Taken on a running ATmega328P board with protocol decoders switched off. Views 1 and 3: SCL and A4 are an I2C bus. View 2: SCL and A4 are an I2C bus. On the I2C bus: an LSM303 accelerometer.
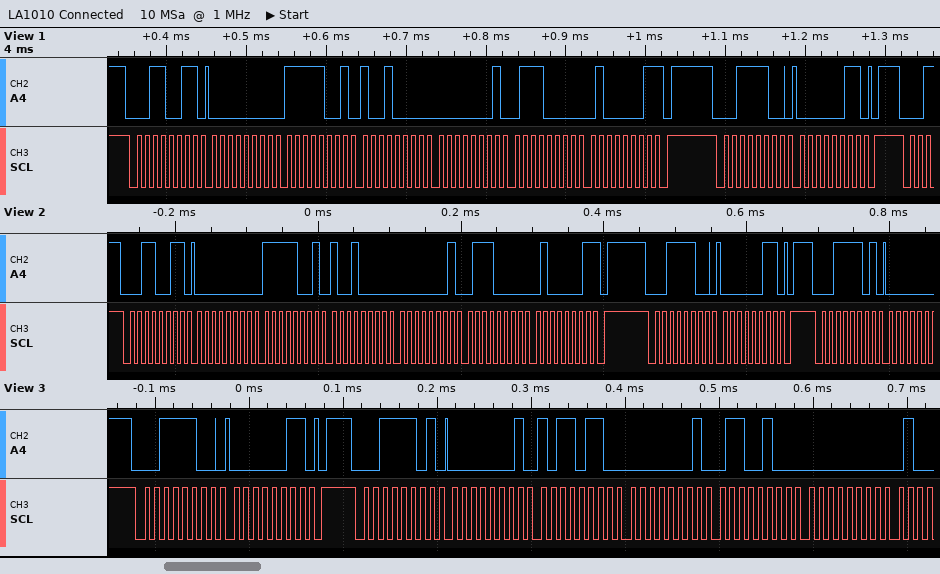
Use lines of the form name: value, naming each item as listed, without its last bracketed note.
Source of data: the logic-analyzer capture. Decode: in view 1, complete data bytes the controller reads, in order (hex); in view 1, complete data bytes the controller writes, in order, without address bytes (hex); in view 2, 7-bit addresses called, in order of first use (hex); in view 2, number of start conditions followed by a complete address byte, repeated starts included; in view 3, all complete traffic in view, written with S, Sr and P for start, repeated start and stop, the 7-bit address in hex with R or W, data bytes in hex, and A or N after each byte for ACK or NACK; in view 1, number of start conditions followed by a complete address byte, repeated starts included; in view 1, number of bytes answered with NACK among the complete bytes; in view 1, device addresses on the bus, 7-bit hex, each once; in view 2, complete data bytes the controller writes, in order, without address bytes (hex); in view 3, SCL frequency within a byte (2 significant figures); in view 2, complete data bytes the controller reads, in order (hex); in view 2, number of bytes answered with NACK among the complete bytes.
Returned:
in view 1, complete data bytes the controller reads, in order: 00 F9 90 01 70 41
in view 1, complete data bytes the controller writes, in order, without address bytes: 03
in view 2, 7-bit addresses called, in order of first use: 0x19 0x1E
in view 2, number of start conditions followed by a complete address byte, repeated starts included: 3
in view 3, all complete traffic in view, written with S, Sr and P for start, repeated start and stop, the 7-bit address in hex with R or W, data bytes in hex, and A or N after each byte for ACK or NACK: S 1EW A 03 A P S 1ER A 01 A B6 A 01 A 64 A 00 A
in view 1, number of start conditions followed by a complete address byte, repeated starts included: 2
in view 1, number of bytes answered with NACK among the complete bytes: 1
in view 1, device addresses on the bus, 7-bit hex, each once: 0x19 0x1E
in view 2, complete data bytes the controller writes, in order, without address bytes: 03
in view 3, SCL frequency within a byte: 100 kHz
in view 2, complete data bytes the controller reads, in order: 00 F9 90 01 70 41
in view 2, number of bytes answered with NACK among the complete bytes: 1
